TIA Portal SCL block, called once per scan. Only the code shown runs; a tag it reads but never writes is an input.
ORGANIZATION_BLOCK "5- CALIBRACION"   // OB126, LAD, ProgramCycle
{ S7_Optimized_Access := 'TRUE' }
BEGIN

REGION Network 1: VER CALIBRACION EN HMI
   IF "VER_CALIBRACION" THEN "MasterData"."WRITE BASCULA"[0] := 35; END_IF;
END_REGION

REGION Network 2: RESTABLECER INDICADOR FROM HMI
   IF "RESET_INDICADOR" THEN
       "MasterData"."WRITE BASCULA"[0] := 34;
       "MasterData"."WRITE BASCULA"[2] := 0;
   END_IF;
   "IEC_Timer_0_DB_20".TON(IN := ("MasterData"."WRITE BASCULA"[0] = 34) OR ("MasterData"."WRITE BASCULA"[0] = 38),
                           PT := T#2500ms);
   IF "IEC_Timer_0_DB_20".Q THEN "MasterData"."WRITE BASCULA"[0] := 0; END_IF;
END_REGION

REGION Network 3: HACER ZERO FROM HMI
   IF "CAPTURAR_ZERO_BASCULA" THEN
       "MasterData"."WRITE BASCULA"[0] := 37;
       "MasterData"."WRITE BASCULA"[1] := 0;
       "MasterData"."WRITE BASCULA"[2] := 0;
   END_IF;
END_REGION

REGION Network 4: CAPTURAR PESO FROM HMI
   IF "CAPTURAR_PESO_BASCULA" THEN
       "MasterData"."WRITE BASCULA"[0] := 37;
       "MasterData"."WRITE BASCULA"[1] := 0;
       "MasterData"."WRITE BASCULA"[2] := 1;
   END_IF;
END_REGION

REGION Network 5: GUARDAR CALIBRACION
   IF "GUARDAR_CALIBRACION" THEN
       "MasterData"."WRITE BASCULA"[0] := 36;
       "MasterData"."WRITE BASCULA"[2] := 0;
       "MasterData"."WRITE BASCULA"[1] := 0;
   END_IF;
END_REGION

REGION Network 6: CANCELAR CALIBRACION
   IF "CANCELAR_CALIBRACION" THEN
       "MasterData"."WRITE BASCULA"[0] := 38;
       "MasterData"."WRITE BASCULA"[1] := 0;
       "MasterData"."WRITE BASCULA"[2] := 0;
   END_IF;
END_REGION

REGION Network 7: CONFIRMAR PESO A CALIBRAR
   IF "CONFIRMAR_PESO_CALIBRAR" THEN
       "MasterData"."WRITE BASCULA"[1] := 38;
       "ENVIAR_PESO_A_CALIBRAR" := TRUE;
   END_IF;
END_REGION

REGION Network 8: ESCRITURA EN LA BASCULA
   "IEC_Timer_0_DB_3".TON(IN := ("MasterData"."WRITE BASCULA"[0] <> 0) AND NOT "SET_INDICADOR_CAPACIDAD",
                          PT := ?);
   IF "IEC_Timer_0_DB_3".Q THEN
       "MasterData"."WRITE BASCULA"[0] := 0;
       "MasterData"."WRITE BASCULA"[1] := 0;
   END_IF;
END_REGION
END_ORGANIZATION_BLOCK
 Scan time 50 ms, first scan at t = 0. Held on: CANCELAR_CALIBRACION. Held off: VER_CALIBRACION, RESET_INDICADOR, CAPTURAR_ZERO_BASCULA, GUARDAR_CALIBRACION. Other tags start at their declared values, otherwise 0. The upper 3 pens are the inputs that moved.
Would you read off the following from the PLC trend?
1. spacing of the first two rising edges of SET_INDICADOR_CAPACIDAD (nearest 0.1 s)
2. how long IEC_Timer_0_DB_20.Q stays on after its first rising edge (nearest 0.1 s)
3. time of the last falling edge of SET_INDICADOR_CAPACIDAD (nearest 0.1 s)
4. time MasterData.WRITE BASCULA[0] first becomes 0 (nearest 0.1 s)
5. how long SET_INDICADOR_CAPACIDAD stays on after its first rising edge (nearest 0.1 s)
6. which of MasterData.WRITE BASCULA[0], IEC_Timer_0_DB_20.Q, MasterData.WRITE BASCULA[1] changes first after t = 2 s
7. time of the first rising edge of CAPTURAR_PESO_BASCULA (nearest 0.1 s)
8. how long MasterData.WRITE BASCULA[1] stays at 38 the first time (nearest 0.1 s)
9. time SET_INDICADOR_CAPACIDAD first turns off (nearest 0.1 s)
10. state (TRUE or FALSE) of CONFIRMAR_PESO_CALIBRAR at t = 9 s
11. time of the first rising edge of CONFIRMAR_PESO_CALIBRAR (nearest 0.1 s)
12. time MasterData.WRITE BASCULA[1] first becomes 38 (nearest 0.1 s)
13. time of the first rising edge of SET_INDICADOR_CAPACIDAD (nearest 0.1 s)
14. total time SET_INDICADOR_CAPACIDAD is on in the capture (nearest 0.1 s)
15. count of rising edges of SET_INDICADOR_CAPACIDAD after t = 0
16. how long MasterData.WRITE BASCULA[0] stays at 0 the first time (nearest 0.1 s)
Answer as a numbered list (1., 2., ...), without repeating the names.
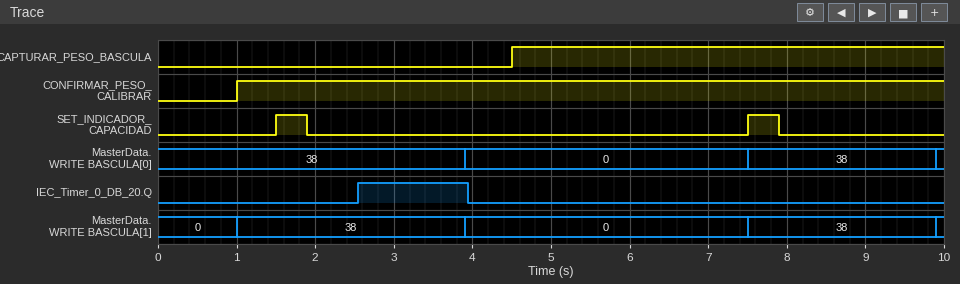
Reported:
1. 6.0 s
2. 1.4 s
3. 7.9 s
4. 3.9 s
5. 0.4 s
6. IEC_Timer_0_DB_20.Q
7. 4.5 s
8. 2.9 s
9. 1.9 s
10. TRUE
11. 1.0 s
12. 1.0 s
13. 1.5 s
14. 0.8 s
15. 2
16. 3.6 s
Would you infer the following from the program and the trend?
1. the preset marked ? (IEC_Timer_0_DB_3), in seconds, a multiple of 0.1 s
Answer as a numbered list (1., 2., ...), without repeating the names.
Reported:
1. 2.0 s
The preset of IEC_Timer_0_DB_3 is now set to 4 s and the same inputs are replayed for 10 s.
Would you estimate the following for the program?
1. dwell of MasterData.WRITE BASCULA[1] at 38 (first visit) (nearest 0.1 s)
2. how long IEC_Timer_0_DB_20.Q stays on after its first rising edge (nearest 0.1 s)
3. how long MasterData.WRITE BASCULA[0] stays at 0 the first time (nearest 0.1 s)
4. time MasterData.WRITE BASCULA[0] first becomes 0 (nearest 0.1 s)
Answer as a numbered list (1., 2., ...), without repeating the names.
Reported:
1. 4.9 s
2. 3.4 s
3. 1.6 s
4. 5.9 s
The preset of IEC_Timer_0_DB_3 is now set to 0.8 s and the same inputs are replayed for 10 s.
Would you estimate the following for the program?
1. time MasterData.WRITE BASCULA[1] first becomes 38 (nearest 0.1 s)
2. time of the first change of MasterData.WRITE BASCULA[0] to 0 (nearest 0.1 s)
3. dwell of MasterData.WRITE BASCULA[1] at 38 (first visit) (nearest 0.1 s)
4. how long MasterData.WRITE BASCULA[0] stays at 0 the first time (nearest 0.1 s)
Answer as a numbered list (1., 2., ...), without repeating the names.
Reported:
1. 1.5 s
2. 0.8 s
3. 1.2 s
4. 0.7 s
